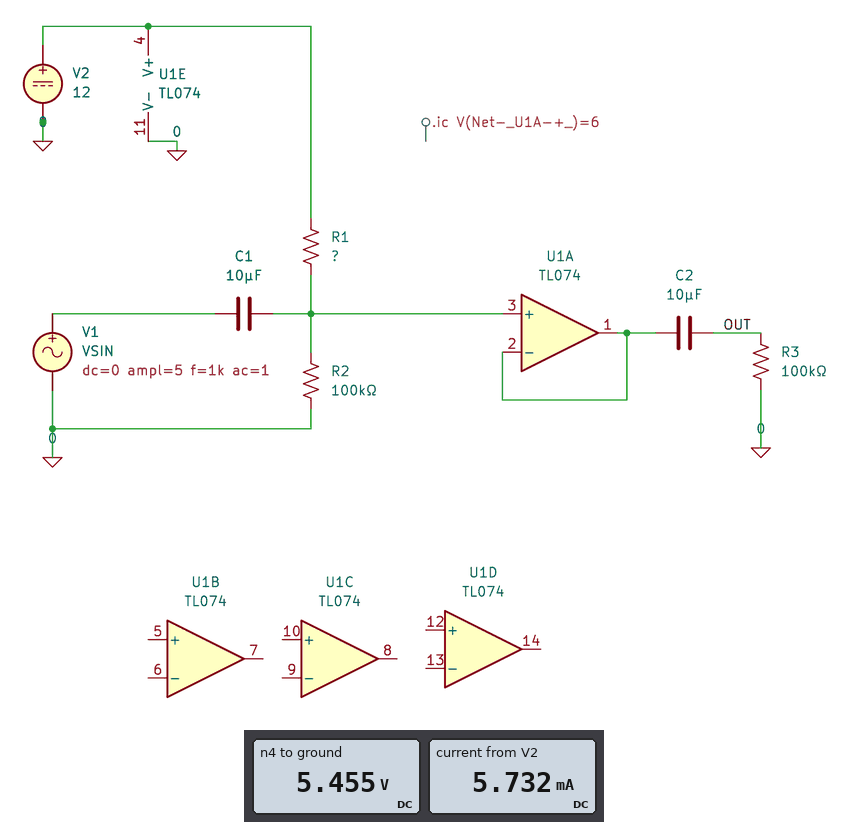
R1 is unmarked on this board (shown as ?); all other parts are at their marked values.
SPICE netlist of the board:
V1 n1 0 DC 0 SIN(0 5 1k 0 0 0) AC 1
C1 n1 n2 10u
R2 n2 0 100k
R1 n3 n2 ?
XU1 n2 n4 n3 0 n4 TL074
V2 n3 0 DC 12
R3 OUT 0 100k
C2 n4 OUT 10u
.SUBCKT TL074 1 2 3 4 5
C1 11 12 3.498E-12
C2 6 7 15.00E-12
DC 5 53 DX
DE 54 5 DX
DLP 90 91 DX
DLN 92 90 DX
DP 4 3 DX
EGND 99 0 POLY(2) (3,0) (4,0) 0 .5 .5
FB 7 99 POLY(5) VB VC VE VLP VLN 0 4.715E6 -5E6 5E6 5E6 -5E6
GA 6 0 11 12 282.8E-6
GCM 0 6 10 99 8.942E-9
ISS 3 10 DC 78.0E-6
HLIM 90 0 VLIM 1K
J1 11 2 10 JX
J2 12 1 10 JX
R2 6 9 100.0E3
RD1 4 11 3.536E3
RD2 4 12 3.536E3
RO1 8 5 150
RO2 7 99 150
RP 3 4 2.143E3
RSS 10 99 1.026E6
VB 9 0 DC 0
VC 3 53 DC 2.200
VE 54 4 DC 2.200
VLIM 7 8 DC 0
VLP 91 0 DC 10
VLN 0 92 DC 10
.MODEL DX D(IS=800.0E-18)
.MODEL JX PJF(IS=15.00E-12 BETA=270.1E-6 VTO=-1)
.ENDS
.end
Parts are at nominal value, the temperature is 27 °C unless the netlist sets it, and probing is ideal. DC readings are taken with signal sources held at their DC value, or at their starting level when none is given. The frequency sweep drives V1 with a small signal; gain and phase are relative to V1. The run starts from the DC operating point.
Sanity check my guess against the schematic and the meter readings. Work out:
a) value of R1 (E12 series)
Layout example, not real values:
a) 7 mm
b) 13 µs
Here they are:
a) 120 kΩ
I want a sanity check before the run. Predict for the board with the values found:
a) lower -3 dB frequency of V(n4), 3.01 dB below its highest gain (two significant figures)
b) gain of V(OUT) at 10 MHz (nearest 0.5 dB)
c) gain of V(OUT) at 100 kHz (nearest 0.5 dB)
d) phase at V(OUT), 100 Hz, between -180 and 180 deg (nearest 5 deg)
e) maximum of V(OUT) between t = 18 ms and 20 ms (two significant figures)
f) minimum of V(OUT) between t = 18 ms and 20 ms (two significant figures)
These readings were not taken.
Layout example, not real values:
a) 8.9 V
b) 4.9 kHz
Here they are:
a) 290 mHz
b) -17.5 dB
c) 0 dB
d) 0 deg
e) 4.9 V
f) -3.9 V
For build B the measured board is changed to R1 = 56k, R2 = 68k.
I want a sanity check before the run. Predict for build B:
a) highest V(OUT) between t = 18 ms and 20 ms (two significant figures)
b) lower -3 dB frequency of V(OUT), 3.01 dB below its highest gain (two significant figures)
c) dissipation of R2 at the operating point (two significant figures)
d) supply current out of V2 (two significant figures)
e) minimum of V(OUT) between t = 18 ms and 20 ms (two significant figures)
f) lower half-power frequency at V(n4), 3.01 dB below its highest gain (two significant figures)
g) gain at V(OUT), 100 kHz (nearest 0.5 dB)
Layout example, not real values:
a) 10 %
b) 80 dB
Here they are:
a) 3.9 V
b) 560 mHz
c) 640 µW
d) 5.8 mA
e) -5.0 V
f) 520 mHz
g) 0 dB
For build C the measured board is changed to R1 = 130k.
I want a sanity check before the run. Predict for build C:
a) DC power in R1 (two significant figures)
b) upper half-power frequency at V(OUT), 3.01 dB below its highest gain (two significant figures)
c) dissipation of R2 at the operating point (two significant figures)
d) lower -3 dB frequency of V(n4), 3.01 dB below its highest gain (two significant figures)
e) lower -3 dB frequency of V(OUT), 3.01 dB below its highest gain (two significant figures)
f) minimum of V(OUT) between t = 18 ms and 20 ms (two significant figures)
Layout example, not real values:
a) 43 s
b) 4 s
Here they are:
a) 350 µW
b) 3.0 MHz
c) 270 µW
d) 280 mHz
e) 350 mHz
f) -3.7 V
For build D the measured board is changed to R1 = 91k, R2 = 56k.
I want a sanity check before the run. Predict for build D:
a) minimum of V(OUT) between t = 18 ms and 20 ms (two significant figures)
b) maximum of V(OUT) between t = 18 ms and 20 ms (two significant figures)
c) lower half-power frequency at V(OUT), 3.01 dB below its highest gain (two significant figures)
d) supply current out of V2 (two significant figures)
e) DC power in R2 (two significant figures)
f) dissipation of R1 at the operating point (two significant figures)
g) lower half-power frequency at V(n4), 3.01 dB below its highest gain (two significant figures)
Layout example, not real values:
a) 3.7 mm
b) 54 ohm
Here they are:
a) -3.0 V
b) 5.8 V
c) 510 mHz
d) 5.8 mA
e) 370 µW
f) 610 µW
g) 460 mHz
